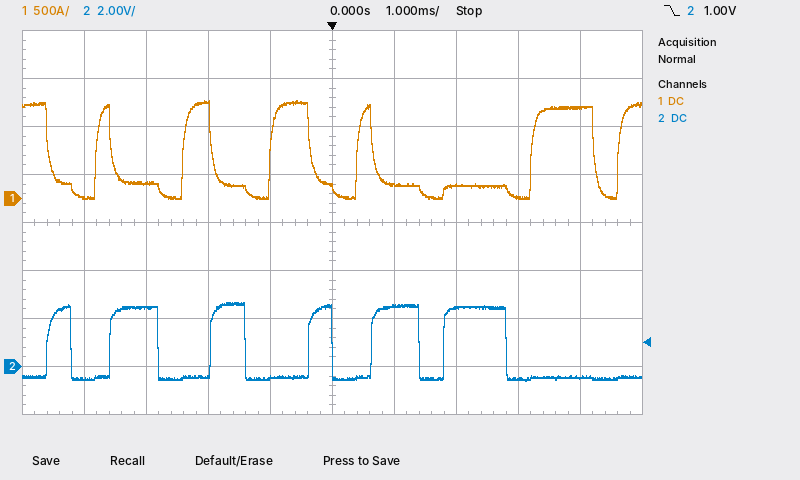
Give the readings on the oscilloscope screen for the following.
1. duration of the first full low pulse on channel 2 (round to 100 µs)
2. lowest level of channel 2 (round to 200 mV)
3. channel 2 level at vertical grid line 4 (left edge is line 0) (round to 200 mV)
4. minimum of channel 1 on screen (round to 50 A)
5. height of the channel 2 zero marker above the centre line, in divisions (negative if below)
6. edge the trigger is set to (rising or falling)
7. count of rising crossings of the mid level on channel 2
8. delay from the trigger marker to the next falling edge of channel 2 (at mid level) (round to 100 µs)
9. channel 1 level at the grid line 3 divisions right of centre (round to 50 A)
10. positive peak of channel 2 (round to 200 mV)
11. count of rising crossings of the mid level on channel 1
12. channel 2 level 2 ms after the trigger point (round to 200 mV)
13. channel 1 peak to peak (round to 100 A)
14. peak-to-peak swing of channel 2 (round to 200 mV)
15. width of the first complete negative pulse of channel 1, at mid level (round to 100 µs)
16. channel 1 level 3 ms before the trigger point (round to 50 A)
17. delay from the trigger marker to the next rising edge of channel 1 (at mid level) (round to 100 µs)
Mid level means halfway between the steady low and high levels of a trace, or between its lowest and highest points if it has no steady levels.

600 µs
-600 mV
-400 mV
0 A
-3.0 div
falling
6
1.4 ms
0 A
2.6 V
6
2.4 V
1.00 kA
3.2 V
800 µs
150 A
400 µs
